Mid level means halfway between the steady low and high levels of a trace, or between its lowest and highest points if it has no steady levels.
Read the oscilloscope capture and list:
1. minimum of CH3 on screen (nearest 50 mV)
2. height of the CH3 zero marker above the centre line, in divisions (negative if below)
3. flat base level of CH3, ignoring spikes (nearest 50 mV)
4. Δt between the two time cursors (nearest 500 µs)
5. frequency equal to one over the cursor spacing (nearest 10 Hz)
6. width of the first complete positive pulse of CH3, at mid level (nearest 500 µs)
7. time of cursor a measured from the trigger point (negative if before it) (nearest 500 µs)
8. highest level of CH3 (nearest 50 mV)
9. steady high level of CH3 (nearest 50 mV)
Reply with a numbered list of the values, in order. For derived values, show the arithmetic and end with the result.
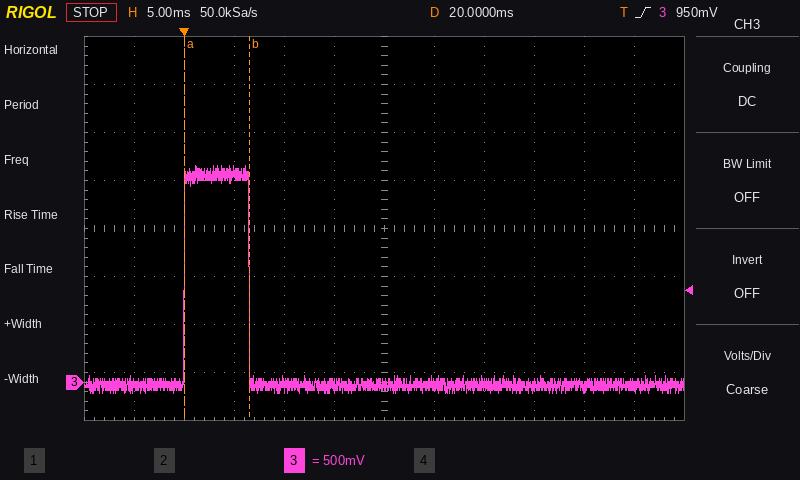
1. -100 mV
2. -3.2 div
3. -50 mV
4. 6.5 ms
5. 1 / 6.5 ms ≈ 150 Hz
6. 6.5 ms
7. 0.0 ms
8. 2.25 V
9. 2.15 V
